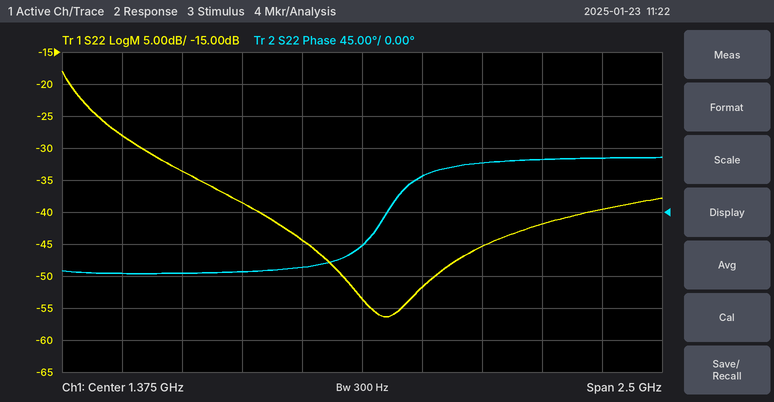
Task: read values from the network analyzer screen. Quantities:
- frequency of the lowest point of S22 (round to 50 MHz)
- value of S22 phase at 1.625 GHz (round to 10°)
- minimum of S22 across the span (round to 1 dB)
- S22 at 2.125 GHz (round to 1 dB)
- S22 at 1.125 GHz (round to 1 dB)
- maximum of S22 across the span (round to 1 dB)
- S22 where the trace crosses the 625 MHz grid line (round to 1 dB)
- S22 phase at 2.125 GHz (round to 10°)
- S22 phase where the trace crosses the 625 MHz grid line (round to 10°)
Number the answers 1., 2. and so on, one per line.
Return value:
1. 1.45 GHz
2. 50°
3. -56 dB
4. -42 dB
5. -44 dB
6. -18 dB
7. -34 dB
8. 70°
9. -90°
